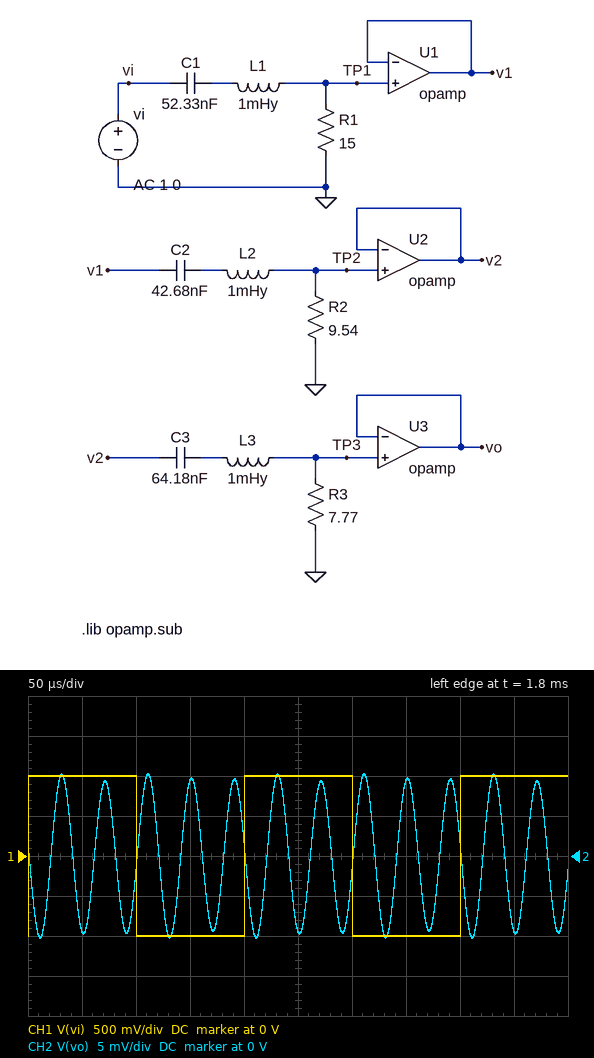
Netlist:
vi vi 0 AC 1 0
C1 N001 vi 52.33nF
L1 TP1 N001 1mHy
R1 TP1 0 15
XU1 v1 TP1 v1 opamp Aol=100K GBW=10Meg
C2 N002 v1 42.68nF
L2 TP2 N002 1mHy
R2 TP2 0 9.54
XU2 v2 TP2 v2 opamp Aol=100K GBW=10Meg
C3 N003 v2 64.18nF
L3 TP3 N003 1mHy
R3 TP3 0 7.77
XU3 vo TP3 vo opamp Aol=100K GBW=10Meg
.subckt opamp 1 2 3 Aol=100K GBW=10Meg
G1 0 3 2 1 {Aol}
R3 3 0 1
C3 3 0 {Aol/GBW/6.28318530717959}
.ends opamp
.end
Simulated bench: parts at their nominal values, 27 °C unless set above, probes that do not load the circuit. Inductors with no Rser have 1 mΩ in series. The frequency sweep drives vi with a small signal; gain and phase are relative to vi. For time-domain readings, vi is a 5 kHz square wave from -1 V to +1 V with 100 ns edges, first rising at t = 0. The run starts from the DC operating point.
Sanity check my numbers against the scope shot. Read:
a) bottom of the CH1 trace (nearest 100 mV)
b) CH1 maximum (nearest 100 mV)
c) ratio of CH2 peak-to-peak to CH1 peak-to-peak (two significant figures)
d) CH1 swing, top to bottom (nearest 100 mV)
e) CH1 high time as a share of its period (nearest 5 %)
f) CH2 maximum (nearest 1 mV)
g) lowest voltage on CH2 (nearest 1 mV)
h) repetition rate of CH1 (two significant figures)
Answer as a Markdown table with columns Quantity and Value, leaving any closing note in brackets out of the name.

| Quantity | Value |
|---|---|
| bottom of the CH1 trace | -1.0 V |
| CH1 maximum | 1.0 V |
| ratio of CH2 peak-to-peak to CH1 peak-to-peak | 0.010 |
| CH1 swing, top to bottom | 2.0 V |
| CH1 high time as a share of its period | 50 % |
| CH2 maximum | 10 mV |
| lowest voltage on CH2 | -10 mV |
| repetition rate of CH1 | 5.0 kHz |
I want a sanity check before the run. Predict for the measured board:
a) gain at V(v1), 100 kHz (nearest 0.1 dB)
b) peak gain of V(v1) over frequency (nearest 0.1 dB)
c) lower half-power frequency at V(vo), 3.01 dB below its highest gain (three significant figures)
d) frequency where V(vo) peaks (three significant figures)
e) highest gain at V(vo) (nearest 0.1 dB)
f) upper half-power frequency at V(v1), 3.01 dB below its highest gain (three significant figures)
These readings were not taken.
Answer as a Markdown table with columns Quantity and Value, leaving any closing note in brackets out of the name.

| Quantity | Value |
|---|---|
| gain at V(v1), 100 kHz | -32.0 dB |
| peak gain of V(v1) over frequency | 0 dB |
| lower half-power frequency at V(vo), 3.01 dB below its highest gain | 19.7 kHz |
| frequency where V(vo) peaks | 22.0 kHz |
| highest gain at V(vo) | -21.4 dB |
| upper half-power frequency at V(v1), 3.01 dB below its highest gain | 23.2 kHz |
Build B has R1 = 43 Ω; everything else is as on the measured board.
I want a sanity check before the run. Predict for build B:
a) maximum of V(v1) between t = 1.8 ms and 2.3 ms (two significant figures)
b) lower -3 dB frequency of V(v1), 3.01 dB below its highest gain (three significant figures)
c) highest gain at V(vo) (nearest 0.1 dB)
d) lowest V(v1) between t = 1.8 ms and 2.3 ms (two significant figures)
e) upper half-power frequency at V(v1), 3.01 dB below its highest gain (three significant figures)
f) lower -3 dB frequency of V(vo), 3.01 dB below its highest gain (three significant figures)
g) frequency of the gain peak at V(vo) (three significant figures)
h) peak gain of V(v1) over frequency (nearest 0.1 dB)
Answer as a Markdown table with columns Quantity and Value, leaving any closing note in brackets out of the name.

| Quantity | Value |
|---|---|
| maximum of V(v1) between t = 1.8 ms and 2.3 ms | 460 mV |
| lower -3 dB frequency of V(v1), 3.01 dB below its highest gain | 18.8 kHz |
| highest gain at V(vo) | -17.8 dB |
| lowest V(v1) between t = 1.8 ms and 2.3 ms | -460 mV |
| upper half-power frequency at V(v1), 3.01 dB below its highest gain | 25.7 kHz |
| lower -3 dB frequency of V(vo), 3.01 dB below its highest gain | 19.5 kHz |
| frequency of the gain peak at V(vo) | 20.0 kHz |
| peak gain of V(v1) over frequency | 0 dB |
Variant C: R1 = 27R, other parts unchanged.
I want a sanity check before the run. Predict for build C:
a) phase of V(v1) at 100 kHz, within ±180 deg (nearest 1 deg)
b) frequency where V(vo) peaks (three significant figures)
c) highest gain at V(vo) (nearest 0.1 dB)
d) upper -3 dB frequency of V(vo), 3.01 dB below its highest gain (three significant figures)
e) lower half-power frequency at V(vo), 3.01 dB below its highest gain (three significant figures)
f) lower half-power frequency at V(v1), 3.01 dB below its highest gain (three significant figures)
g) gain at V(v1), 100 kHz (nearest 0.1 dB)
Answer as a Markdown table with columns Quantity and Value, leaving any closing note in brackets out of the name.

| Quantity | Value |
|---|---|
| phase of V(v1) at 100 kHz, within ±180 deg | -88 deg |
| frequency where V(vo) peaks | 20.1 kHz |
| highest gain at V(vo) | -19.2 dB |
| upper -3 dB frequency of V(vo), 3.01 dB below its highest gain | 24.8 kHz |
| lower half-power frequency at V(vo), 3.01 dB below its highest gain | 19.5 kHz |
| lower half-power frequency at V(v1), 3.01 dB below its highest gain | 20.0 kHz |
| gain at V(v1), 100 kHz | -26.9 dB |
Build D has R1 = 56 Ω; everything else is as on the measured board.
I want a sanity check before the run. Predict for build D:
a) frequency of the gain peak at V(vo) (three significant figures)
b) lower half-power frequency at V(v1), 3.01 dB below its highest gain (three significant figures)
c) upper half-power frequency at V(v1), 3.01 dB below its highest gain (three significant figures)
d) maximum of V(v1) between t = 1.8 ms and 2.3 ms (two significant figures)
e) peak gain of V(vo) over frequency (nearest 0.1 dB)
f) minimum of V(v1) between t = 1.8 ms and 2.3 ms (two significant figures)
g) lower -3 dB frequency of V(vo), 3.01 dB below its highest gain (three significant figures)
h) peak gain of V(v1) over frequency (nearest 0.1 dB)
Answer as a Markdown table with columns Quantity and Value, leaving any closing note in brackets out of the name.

| Quantity | Value |
|---|---|
| frequency of the gain peak at V(vo) | 20.0 kHz |
| lower half-power frequency at V(v1), 3.01 dB below its highest gain | 18.0 kHz |
| upper half-power frequency at V(v1), 3.01 dB below its highest gain | 26.9 kHz |
| maximum of V(v1) between t = 1.8 ms and 2.3 ms | 580 mV |
| peak gain of V(vo) over frequency | -17.3 dB |
| minimum of V(v1) between t = 1.8 ms and 2.3 ms | -580 mV |
| lower -3 dB frequency of V(vo), 3.01 dB below its highest gain | 19.5 kHz |
| peak gain of V(v1) over frequency | 0 dB |
